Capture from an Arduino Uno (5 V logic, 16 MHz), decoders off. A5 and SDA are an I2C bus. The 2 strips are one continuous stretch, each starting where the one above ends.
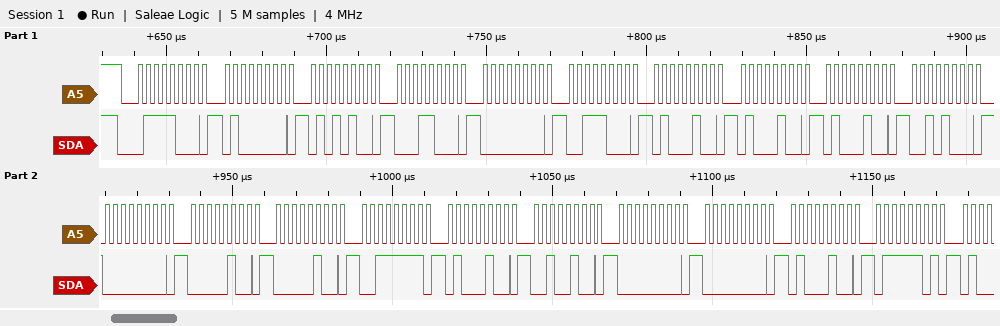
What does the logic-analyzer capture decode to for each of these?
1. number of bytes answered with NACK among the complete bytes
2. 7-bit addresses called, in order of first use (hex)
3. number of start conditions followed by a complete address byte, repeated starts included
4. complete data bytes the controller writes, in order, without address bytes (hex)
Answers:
0
0x3C
1
40 54 18 00 38 44 44 44 28 00 04 04 3F 44 24 00 00 44 7D
